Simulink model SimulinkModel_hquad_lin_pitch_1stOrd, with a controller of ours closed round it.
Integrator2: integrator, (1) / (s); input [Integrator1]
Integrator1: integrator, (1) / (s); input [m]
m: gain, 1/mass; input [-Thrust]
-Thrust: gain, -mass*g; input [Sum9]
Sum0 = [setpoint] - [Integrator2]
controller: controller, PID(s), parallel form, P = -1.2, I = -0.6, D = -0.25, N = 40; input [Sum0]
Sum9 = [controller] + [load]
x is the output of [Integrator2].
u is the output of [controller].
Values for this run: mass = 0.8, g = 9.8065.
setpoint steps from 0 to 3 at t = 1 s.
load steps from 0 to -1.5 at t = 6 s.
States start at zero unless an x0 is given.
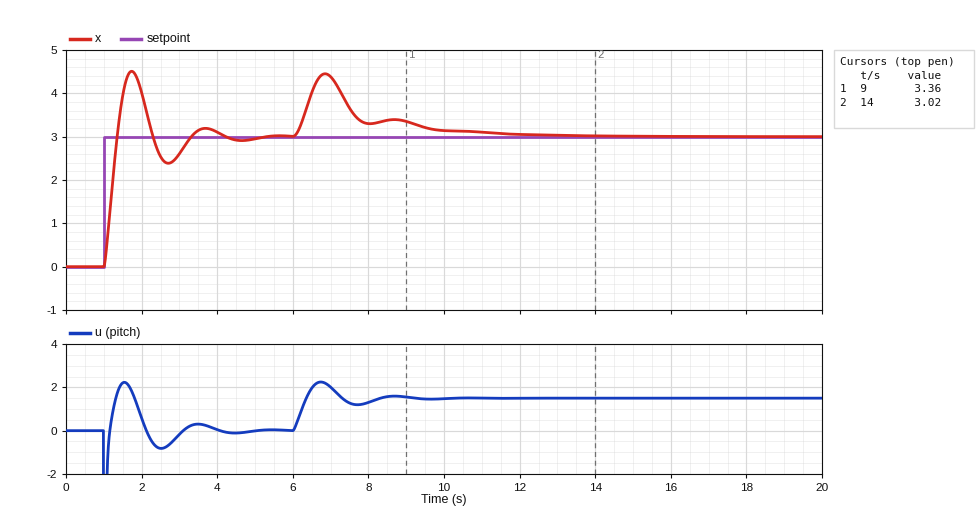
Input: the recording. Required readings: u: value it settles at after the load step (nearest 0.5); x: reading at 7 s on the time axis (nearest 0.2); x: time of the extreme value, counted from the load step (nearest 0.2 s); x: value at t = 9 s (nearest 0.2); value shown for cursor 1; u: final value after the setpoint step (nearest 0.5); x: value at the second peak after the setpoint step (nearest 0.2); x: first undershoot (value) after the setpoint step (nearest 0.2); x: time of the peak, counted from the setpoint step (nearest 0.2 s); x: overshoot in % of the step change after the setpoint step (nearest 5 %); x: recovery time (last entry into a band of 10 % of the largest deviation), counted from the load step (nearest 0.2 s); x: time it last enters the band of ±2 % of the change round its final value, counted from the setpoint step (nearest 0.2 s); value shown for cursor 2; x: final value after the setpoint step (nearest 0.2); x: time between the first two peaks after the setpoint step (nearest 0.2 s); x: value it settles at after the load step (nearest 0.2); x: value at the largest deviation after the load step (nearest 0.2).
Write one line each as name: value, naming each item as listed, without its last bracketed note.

u: value it settles at after the load step: 1.5
x: reading at 7 s on the time axis: 4.4
x: time of the extreme value, counted from the load step: 0.8 s
x: value at t = 9 s: 3.4
value shown for cursor 1: 3.36
u: final value after the setpoint step: 0.0
x: value at the second peak after the setpoint step: 3.2
x: first undershoot (value) after the setpoint step: 2.4
x: time of the peak, counted from the setpoint step: 0.8 s
x: overshoot in % of the step change after the setpoint step: 50 %
x: recovery time (last entry into a band of 10 % of the largest deviation), counted from the load step: 4.0 s
x: time it last enters the band of ±2 % of the change round its final value, counted from the setpoint step: 4.0 s
value shown for cursor 2: 3.02
x: final value after the setpoint step: 3.0
x: time between the first two peaks after the setpoint step: 2.0 s
x: value it settles at after the load step: 3.0
x: value at the largest deviation after the load step: 4.4
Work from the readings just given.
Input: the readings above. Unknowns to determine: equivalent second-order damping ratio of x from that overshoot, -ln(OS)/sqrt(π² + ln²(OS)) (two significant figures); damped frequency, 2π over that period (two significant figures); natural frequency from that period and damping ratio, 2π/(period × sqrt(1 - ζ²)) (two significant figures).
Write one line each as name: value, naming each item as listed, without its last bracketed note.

equivalent second-order damping ratio of x from that overshoot, -ln(OS)/sqrt(π² + ln²(OS)): 0.22
damped frequency, 2π over that period: 3.1 rad/s
natural frequency from that period and damping ratio, 2π/(period × sqrt(1 - ζ²)): 3.2 rad/s
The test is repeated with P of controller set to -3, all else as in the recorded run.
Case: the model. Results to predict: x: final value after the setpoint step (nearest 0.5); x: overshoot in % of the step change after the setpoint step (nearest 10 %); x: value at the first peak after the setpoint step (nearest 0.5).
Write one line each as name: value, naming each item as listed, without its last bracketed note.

x: final value after the setpoint step: 3.0
x: overshoot in % of the step change after the setpoint step: 60 %
x: value at the first peak after the setpoint step: 5.0
